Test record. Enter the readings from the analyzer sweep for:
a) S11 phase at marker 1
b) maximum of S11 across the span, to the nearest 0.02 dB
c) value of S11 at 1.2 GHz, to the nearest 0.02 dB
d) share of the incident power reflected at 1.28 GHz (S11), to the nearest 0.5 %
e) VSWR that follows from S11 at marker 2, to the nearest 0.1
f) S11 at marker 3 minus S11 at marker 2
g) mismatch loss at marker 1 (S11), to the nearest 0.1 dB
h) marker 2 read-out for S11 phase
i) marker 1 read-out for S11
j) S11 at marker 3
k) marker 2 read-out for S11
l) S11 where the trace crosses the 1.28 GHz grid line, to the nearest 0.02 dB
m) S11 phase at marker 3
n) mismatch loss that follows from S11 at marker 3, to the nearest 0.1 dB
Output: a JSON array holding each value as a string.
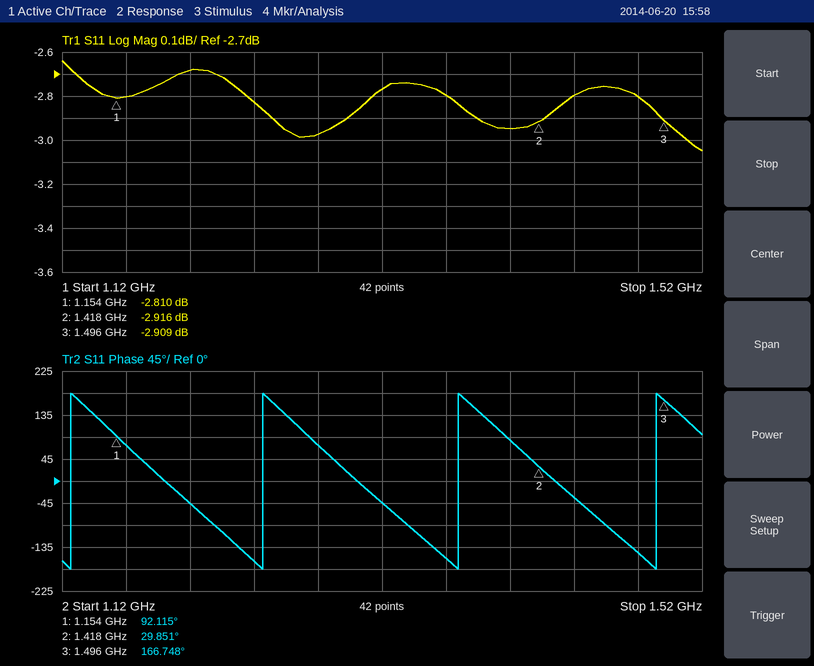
["92.115°", "-2.64 dB", "-2.68 dB", "50.5 %", "6.0", "0.007 dB", "3.2 dB", "29.851°", "-2.810 dB", "-2.909 dB", "-2.916 dB", "-2.98 dB", "166.748°", "3.1 dB"]
